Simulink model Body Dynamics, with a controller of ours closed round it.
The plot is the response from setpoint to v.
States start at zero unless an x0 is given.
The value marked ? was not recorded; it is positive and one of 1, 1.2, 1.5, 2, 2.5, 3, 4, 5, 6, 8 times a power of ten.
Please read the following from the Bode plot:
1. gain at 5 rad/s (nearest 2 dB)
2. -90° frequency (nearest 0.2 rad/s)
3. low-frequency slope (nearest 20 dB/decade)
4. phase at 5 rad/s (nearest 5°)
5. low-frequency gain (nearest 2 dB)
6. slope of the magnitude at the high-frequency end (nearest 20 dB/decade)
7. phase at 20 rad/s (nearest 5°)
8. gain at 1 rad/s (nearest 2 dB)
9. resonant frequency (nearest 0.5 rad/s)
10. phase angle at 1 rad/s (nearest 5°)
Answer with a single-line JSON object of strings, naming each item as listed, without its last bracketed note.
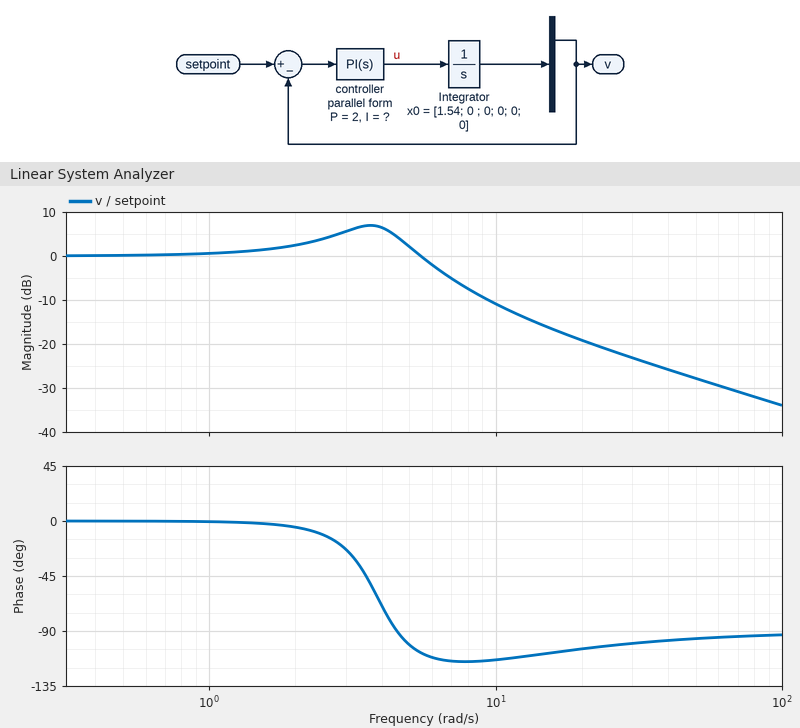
{"gain at 5 rad/s": "2 dB", "-90° frequency": "4.6 rad/s", "low-frequency slope": "0 dB/decade", "phase at 5 rad/s": "-100°", "low-frequency gain": "0 dB", "slope of the magnitude at the high-frequency end": "-20 dB/decade", "phase at 20 rad/s": "-105°", "gain at 1 rad/s": "0 dB", "resonant frequency": "3.5 rad/s", "phase angle at 1 rad/s": "0°"}
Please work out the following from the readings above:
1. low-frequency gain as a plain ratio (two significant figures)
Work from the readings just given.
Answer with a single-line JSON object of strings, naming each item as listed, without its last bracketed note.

{"low-frequency gain as a plain ratio": "1.0"}
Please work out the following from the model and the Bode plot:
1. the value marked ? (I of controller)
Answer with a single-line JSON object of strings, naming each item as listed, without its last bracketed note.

{"the value marked ?": "15"}
